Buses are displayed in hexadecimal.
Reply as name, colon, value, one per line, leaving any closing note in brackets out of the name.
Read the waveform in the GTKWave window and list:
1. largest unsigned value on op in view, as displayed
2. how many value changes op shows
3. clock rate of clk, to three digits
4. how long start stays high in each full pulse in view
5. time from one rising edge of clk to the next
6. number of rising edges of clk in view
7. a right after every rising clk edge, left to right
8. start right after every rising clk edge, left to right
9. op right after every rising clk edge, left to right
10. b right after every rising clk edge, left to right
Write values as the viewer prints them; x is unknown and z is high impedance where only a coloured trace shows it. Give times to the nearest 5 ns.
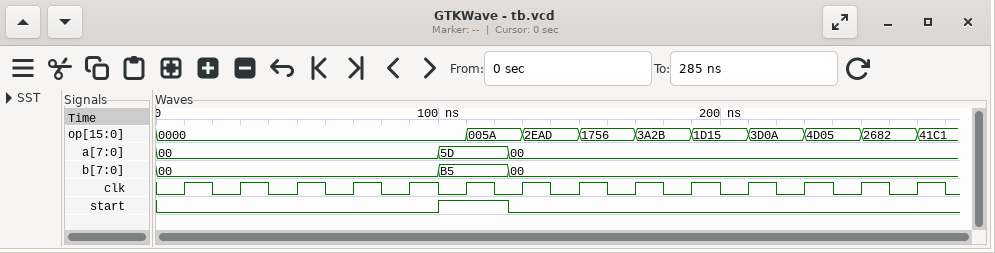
largest unsigned value on op in view, as displayed: 4D05
how many value changes op shows: 9
clock rate of clk, to three digits: 50.0 MHz
how long start stays high in each full pulse in view: 25 ns
time from one rising edge of clk to the next: 20 ns
number of rising edges of clk in view: 14
a right after every rising clk edge, left to right: 00, 00, 00, 00, 00, 5D, 00, 00, 00, 00, 00, 00, 00, 00
start right after every rising clk edge, left to right: 0 0 0 0 0 1 0 0 0 0 0 0 0 0
op right after every rising clk edge, left to right: 0000, 0000, 0000, 0000, 0000, 005A, 2EAD, 1756, 3A2B, 1D15, 3D0A, 4D05, 2682, 41C1
b right after every rising clk edge, left to right: 00, 00, 00, 00, 00, B5, 00, 00, 00, 00, 00, 00, 00, 00
